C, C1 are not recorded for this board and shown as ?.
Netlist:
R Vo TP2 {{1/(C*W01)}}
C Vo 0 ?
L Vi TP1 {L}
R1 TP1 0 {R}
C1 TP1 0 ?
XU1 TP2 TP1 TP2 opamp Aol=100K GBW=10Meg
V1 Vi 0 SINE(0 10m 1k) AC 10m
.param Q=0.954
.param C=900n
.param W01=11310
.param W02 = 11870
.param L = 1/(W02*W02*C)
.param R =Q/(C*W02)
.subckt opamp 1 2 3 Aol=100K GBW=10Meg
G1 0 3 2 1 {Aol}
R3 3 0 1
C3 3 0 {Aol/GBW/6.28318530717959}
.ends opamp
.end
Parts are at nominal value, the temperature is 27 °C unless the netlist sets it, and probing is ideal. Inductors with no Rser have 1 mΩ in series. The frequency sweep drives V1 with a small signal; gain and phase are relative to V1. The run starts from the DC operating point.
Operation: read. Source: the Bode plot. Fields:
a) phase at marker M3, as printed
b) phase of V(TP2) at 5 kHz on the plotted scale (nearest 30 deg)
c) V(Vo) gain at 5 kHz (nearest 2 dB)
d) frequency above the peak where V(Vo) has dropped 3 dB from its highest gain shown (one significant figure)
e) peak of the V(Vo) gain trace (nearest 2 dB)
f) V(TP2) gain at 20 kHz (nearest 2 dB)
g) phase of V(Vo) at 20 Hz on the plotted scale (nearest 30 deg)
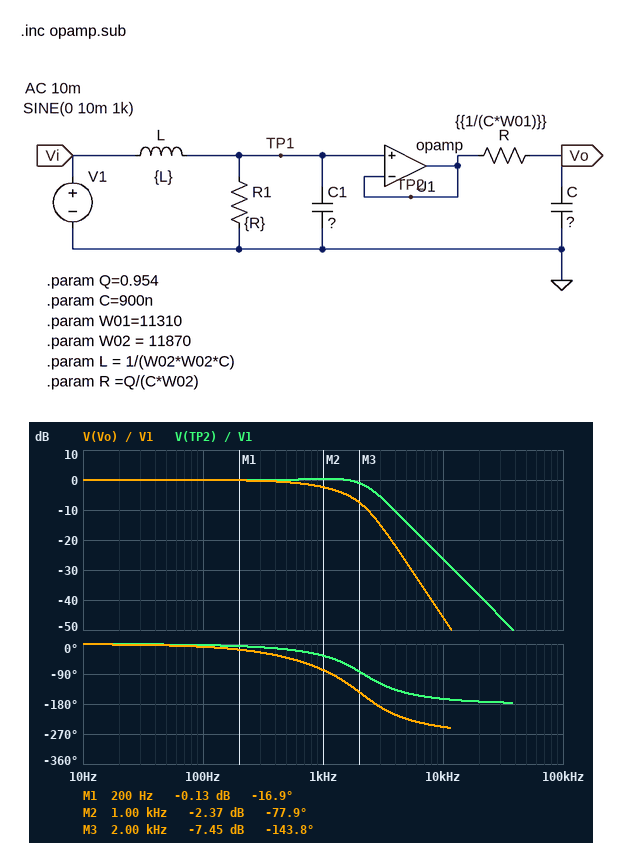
-143.8 deg
-150 deg
-28 dB
1 kHz
0 dB
-38 dB
0 deg
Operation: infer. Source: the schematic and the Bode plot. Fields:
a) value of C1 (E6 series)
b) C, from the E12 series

680 nF
1.5 µF
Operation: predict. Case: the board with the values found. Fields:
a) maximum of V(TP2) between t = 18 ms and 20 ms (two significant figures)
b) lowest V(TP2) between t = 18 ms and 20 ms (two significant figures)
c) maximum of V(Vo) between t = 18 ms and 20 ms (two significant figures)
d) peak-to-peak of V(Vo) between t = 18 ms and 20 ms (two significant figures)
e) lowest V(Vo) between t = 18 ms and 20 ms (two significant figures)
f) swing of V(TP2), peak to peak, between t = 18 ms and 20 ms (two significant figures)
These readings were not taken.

10 mV
-10 mV
7.6 mV
15 mV
-7.6 mV
21 mV
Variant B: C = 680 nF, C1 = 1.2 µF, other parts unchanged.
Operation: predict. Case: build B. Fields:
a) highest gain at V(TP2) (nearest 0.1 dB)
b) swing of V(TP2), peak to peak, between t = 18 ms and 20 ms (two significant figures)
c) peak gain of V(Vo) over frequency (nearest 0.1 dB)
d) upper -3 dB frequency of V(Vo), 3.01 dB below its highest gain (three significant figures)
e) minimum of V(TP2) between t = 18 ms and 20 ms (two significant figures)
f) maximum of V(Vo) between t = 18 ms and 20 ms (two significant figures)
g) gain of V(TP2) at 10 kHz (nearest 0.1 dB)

1.8 dB
24 mV
0.9 dB
1.80 kHz
-12 mV
11 mV
-31.3 dB
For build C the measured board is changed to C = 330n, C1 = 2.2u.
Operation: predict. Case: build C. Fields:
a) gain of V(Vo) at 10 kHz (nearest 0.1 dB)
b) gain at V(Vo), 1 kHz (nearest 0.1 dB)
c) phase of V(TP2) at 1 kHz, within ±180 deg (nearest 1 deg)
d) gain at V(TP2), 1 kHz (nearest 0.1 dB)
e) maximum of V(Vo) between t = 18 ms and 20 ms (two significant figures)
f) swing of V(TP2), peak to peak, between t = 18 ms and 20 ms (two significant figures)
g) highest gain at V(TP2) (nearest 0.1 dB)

-43.7 dB
3.7 dB
-60 deg
3.9 dB
15 mV
31 mV
4.0 dB
